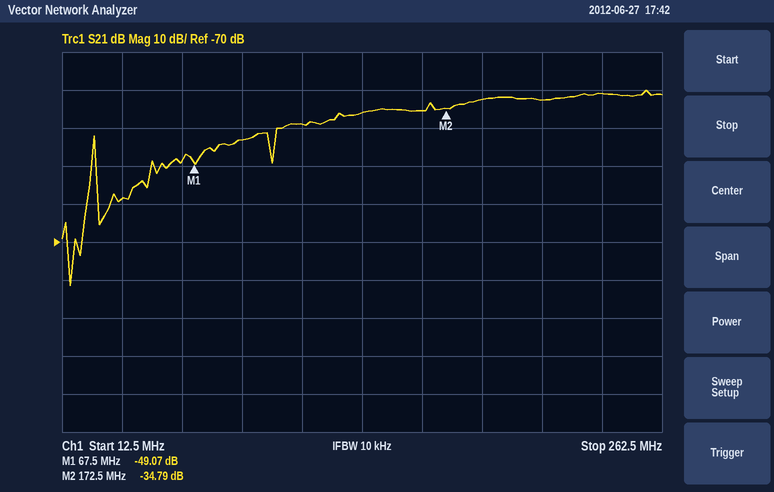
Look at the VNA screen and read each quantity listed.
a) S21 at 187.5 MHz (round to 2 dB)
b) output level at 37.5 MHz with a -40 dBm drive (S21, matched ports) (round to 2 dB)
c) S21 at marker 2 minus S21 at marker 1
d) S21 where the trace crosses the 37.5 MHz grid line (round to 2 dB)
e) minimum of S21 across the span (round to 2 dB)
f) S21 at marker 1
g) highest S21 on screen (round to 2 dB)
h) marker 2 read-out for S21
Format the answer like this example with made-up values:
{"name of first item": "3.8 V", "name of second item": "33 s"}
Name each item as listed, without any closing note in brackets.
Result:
{"S21 at 187.5 MHz": "-32 dB", "output level at 37.5 MHz with a -40 dBm drive (S21, matched ports)": "-98 dBm", "S21 at marker 2 minus S21 at marker 1": "14.28 dB", "S21 where the trace crosses the 37.5 MHz grid line": "-58 dB", "minimum of S21 across the span": "-82 dB", "S21 at marker 1": "-49.07 dB", "highest S21 on screen": "-30 dB", "marker 2 read-out for S21": "-34.79 dB"}
